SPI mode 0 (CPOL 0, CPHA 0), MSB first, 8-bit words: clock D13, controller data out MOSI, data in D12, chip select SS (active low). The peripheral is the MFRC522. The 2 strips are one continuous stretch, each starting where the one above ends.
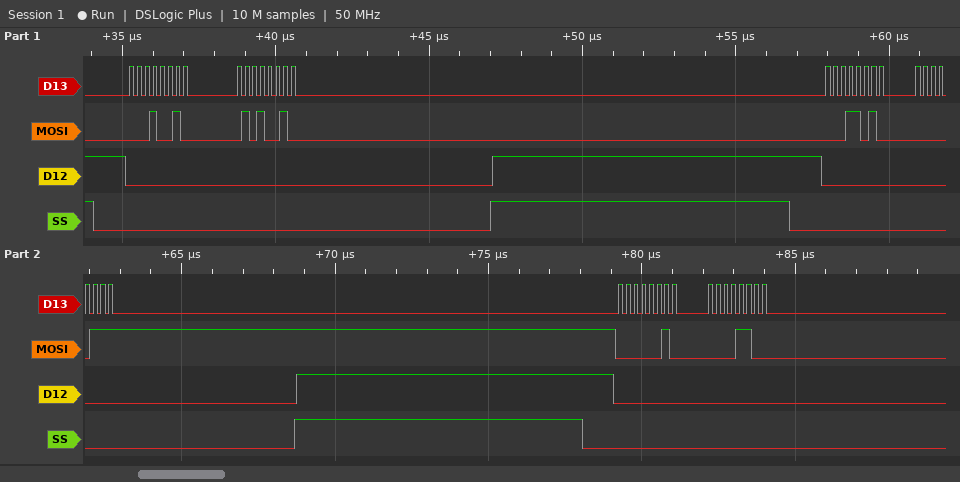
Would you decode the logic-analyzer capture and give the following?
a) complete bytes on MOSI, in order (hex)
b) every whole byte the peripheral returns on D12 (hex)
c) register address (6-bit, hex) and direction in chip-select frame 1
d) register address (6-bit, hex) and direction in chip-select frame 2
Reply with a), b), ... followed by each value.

a) 12 52 1A 07 02 0C
b) 00 00 00 00 00 00
c) 0x09 write
d) 0x0D write
